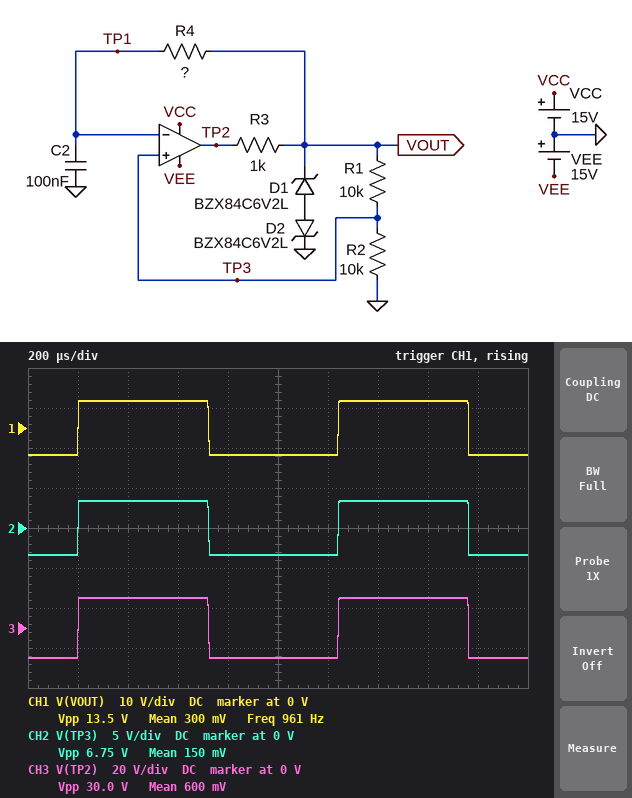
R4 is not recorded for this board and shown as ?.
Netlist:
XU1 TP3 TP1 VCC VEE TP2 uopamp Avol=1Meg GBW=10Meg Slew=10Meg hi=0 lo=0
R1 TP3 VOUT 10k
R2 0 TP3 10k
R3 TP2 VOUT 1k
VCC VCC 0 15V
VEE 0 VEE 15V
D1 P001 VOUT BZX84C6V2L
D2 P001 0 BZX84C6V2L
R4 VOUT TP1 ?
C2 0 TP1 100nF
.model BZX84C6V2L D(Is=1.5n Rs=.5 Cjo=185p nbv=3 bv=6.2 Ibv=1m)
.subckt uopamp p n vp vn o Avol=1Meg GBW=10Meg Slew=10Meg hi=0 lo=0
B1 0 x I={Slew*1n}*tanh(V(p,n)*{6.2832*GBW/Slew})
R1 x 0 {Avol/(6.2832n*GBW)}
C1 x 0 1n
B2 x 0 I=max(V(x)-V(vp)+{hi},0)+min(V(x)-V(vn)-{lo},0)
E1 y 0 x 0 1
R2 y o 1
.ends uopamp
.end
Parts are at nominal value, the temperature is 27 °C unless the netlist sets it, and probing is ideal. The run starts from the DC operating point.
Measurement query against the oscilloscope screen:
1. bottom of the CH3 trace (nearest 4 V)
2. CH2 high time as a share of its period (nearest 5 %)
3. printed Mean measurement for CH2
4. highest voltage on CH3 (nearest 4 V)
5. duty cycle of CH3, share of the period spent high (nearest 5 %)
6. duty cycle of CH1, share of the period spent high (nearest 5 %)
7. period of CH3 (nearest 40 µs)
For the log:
-16 V
50 %
150 mV
16 V
50 %
50 %
1.04 ms
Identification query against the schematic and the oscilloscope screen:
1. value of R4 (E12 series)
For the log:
4.7 kΩ
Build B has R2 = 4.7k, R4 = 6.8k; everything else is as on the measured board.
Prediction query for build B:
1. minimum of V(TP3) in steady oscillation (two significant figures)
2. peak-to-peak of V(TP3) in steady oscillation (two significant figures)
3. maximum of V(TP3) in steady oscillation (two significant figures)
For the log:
-2.2 V
4.3 V
2.2 V
